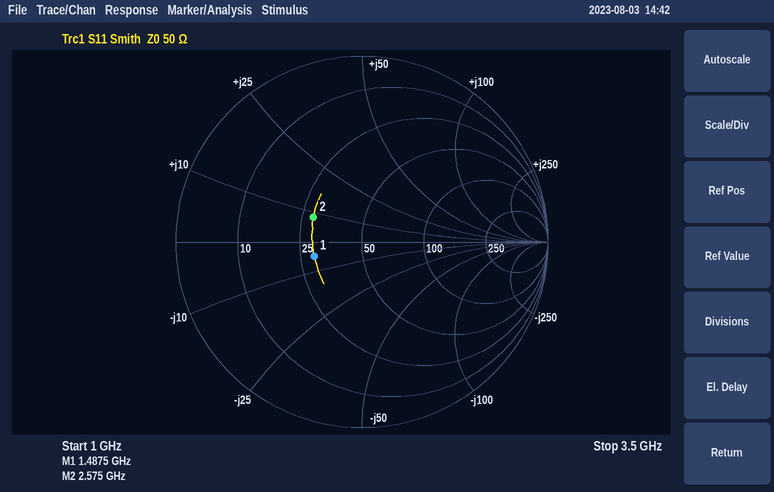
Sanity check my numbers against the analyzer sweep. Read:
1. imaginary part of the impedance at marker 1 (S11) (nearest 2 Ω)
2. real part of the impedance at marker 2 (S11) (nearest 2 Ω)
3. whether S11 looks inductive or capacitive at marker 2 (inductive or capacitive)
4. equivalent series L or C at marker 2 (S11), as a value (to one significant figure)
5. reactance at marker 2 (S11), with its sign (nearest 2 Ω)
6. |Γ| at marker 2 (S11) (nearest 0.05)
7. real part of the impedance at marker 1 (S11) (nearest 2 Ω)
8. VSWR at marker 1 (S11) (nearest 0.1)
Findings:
-4 Ω
28 Ω
inductive
500 pH
+8 Ω
0.30
30 Ω
1.7
